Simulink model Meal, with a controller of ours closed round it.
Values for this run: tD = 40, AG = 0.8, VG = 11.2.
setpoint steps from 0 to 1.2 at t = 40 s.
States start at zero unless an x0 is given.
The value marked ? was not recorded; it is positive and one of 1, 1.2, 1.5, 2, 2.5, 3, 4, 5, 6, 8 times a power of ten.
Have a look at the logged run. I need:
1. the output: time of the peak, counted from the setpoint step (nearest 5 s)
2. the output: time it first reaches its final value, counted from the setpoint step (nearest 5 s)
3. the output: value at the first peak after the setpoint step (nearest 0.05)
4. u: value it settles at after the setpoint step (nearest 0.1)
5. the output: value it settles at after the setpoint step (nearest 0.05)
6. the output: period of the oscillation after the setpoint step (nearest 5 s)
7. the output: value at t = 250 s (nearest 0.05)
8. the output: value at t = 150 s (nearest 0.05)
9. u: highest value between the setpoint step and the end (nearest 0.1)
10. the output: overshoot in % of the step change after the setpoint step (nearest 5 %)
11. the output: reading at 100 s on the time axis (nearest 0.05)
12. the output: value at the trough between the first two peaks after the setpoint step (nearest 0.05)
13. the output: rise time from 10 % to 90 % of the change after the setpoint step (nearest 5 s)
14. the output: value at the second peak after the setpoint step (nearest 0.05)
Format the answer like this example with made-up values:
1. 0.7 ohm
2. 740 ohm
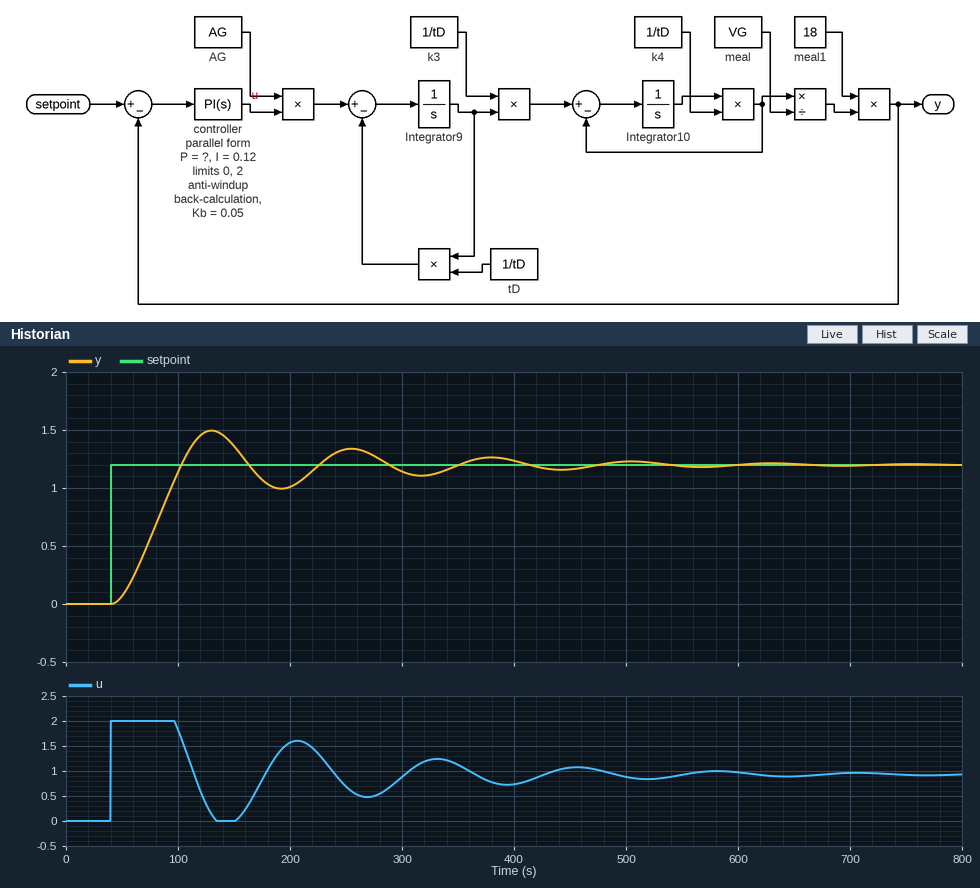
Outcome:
1. 90 s
2. 65 s
3. 1.50
4. 0.9
5. 1.20
6. 125 s
7. 1.35
8. 1.35
9. 2.0
10. 25 %
11. 1.15
12. 1.00
13. 45 s
14. 1.35
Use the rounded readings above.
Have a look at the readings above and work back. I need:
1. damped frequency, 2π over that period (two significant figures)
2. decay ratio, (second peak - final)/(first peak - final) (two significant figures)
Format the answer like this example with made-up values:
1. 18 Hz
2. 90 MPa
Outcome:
1. 0.050 rad/s
2. 0.50
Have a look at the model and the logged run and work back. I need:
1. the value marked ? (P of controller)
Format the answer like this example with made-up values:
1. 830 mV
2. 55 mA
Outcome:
1. 3
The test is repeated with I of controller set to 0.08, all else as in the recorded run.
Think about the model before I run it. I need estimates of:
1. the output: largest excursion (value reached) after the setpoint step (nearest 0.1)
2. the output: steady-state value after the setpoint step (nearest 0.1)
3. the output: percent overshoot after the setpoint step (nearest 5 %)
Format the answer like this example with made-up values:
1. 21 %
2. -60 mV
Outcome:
1. 1.4
2. 1.2
3. 15 %
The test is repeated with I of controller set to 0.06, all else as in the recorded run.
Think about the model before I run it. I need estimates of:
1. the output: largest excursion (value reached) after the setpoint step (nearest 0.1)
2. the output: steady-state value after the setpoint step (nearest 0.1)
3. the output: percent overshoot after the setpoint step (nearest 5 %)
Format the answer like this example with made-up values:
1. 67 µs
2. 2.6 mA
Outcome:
1. 1.3
2. 1.2
3. 10 %
